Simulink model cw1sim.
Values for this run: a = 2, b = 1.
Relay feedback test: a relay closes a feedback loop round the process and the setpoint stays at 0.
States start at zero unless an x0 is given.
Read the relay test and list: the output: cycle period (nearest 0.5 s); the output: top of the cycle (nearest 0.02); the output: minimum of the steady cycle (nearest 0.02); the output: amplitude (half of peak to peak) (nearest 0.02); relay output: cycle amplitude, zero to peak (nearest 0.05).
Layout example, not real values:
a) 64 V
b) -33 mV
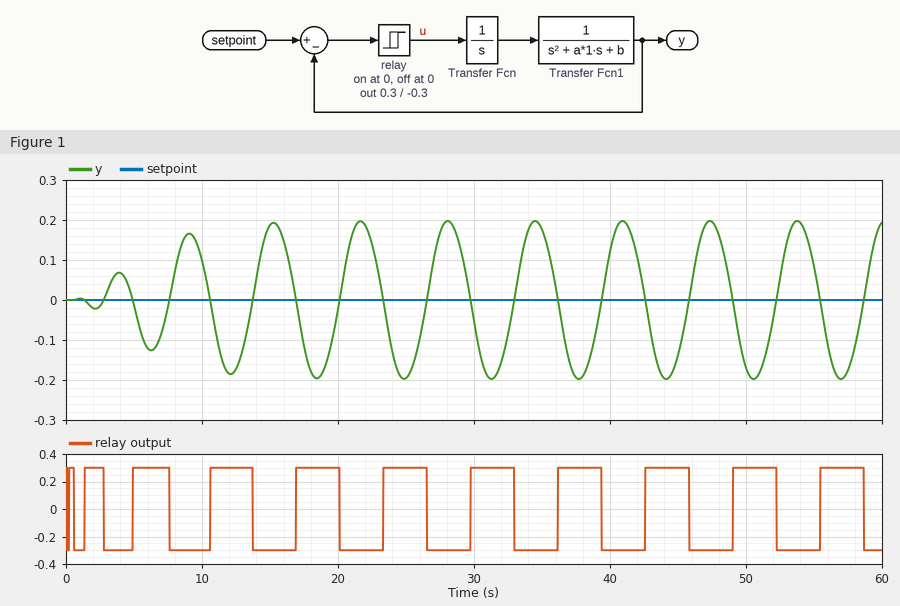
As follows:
a) 6.5 s
b) 0.20
c) -0.20
d) 0.20
e) 0.30
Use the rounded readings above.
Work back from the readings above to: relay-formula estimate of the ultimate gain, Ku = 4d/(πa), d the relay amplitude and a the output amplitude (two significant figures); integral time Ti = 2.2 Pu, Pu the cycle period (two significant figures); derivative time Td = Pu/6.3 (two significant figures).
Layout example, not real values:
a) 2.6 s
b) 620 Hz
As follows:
a) 1.9
b) 14 s
c) 1.0 s
